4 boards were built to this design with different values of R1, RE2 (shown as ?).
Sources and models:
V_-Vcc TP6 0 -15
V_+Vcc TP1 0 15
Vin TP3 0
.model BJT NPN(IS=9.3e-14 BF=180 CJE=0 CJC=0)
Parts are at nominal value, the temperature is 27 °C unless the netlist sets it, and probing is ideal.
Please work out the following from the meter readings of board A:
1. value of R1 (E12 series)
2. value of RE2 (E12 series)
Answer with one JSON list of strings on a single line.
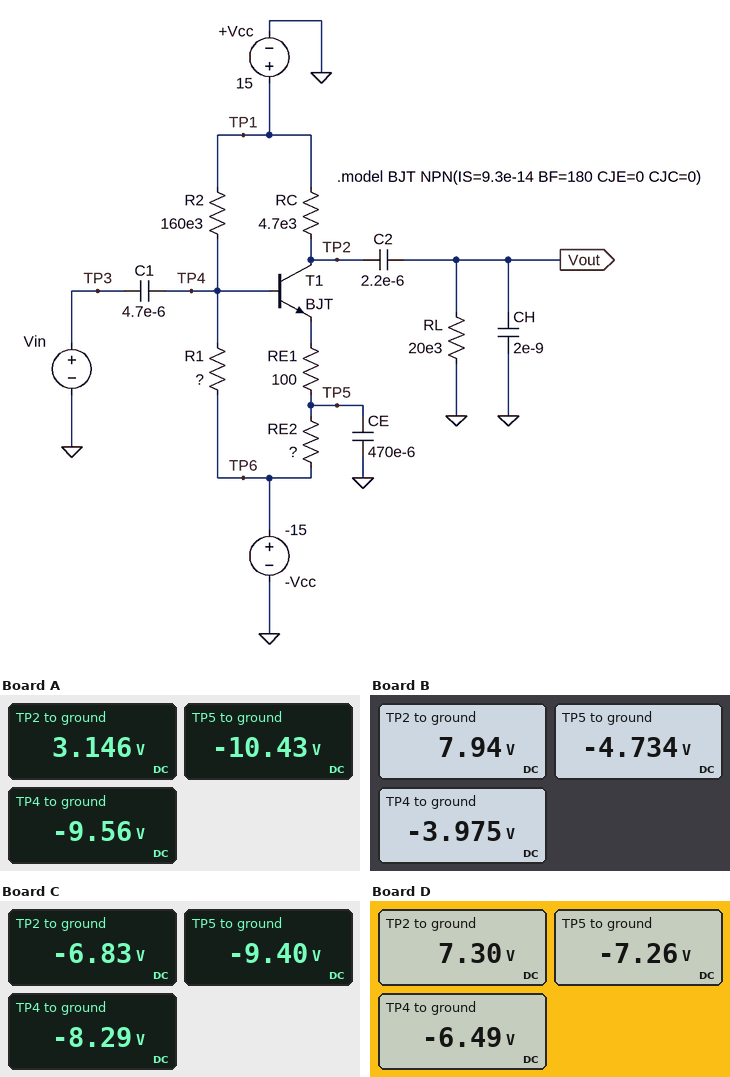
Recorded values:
["39 kΩ", "1.8 kΩ"]
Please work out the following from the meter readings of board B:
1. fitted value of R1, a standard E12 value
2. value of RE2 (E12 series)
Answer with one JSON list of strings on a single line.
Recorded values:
["100 kΩ", "6.8 kΩ"]
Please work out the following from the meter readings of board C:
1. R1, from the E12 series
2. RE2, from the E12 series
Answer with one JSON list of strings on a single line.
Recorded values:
["56 kΩ", "1.2 kΩ"]
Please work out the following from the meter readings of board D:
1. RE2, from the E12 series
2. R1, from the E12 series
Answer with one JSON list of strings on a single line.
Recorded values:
["4.7 kΩ", "68 kΩ"]
